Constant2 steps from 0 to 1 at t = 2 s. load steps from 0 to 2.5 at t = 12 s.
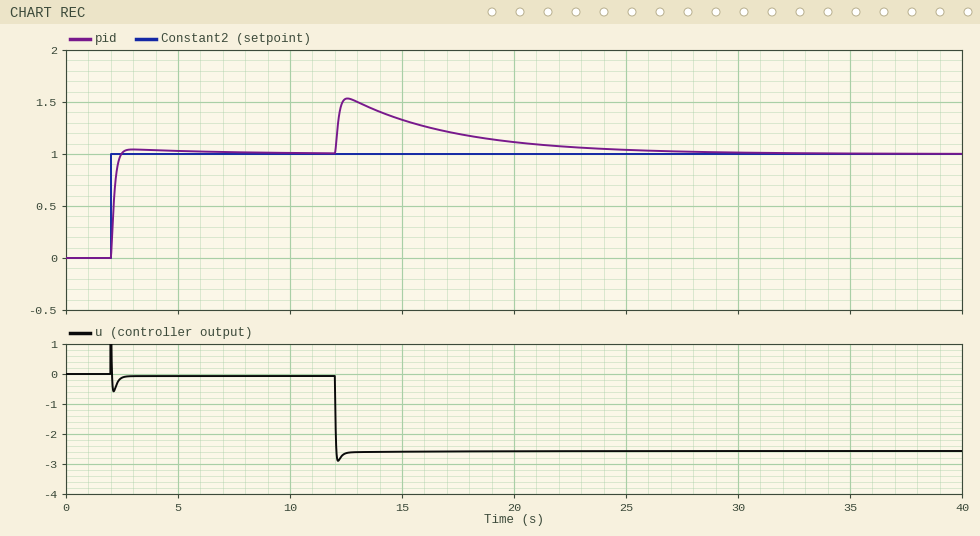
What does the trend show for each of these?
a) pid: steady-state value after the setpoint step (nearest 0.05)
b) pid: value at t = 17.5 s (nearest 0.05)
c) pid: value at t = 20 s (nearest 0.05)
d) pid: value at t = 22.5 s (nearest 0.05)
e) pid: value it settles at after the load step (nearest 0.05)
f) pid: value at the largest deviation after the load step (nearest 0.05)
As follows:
1.00
1.20
1.10
1.05
1.00
1.55
